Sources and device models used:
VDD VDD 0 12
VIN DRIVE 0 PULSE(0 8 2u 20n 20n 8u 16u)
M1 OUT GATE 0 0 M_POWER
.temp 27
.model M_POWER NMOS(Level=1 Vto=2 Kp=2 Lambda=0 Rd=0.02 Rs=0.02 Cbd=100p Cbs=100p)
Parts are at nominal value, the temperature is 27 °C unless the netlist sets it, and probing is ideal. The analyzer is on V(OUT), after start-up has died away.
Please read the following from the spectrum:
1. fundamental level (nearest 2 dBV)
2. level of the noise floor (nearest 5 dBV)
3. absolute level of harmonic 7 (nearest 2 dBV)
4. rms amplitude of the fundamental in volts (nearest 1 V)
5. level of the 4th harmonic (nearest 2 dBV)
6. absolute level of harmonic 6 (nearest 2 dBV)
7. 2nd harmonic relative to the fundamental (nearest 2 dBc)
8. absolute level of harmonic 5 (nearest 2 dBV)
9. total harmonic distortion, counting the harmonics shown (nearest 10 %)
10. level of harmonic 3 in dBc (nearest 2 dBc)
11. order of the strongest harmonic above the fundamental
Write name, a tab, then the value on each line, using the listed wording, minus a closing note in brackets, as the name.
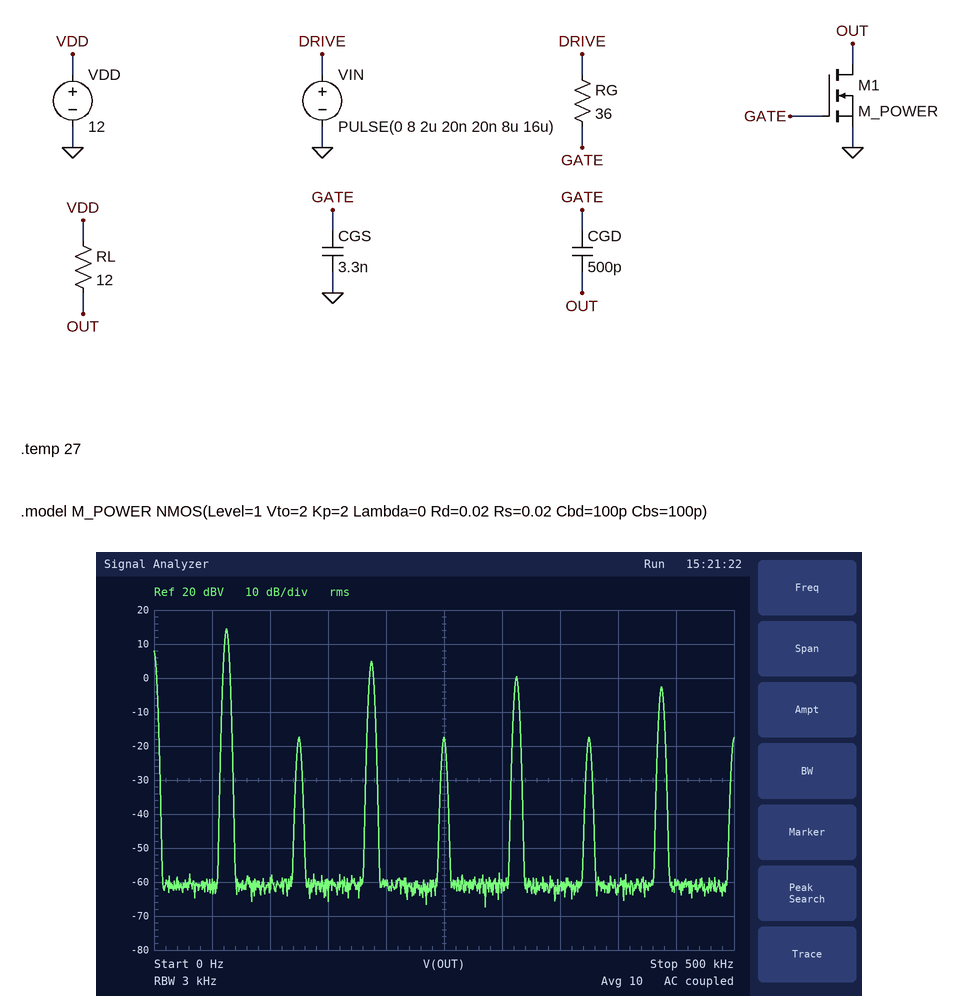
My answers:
fundamental level	14 dBV
level of the noise floor	-60 dBV
absolute level of harmonic 7	-2 dBV
rms amplitude of the fundamental in volts	5 V
level of the 4th harmonic	-18 dBV
absolute level of harmonic 6	-18 dBV
2nd harmonic relative to the fundamental	-32 dBc
absolute level of harmonic 5	0 dBV
total harmonic distortion, counting the harmonics shown	40 %
level of harmonic 3 in dBc	-10 dBc
order of the strongest harmonic above the fundamental	3
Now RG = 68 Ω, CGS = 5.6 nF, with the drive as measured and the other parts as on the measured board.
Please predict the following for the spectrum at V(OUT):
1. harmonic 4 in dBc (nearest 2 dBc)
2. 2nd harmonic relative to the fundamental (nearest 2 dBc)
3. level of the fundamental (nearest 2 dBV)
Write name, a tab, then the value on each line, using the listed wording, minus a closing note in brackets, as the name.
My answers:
harmonic 4 in dBc	-24 dBc
2nd harmonic relative to the fundamental	-24 dBc
level of the fundamental	14 dBV
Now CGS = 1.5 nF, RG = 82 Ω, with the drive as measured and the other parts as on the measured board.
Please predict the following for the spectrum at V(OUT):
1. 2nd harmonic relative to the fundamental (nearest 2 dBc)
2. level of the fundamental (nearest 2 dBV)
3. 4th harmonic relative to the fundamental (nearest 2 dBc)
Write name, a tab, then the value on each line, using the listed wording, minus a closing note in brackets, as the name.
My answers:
2nd harmonic relative to the fundamental	-30 dBc
level of the fundamental	14 dBV
4th harmonic relative to the fundamental	-30 dBc
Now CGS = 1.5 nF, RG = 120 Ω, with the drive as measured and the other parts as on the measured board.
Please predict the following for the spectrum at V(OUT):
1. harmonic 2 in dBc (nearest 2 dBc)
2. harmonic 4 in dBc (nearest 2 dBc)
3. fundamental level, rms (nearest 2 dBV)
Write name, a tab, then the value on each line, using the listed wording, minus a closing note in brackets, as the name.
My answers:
harmonic 2 in dBc	-26 dBc
harmonic 4 in dBc	-26 dBc
fundamental level, rms	14 dBV
